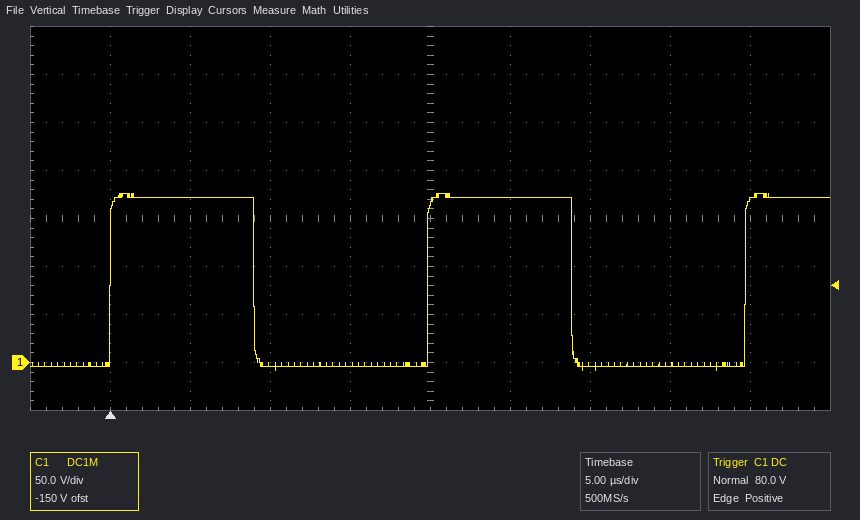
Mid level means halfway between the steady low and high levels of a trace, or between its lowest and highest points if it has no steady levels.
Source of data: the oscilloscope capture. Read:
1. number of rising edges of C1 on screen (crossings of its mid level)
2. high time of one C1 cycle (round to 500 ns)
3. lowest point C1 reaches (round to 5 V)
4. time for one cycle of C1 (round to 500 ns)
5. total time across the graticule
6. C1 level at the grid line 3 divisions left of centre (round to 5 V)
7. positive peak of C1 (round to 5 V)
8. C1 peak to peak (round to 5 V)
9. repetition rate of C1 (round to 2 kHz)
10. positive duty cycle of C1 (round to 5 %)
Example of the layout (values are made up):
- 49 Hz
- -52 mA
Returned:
- 3
- 9.0 µs
- -10 V
- 20.0 µs
- 50 µs
- 170 V
- 175 V
- 185 V
- 50 kHz
- 45 %
